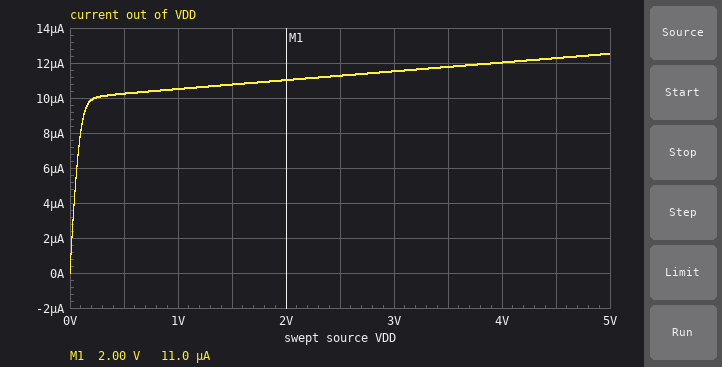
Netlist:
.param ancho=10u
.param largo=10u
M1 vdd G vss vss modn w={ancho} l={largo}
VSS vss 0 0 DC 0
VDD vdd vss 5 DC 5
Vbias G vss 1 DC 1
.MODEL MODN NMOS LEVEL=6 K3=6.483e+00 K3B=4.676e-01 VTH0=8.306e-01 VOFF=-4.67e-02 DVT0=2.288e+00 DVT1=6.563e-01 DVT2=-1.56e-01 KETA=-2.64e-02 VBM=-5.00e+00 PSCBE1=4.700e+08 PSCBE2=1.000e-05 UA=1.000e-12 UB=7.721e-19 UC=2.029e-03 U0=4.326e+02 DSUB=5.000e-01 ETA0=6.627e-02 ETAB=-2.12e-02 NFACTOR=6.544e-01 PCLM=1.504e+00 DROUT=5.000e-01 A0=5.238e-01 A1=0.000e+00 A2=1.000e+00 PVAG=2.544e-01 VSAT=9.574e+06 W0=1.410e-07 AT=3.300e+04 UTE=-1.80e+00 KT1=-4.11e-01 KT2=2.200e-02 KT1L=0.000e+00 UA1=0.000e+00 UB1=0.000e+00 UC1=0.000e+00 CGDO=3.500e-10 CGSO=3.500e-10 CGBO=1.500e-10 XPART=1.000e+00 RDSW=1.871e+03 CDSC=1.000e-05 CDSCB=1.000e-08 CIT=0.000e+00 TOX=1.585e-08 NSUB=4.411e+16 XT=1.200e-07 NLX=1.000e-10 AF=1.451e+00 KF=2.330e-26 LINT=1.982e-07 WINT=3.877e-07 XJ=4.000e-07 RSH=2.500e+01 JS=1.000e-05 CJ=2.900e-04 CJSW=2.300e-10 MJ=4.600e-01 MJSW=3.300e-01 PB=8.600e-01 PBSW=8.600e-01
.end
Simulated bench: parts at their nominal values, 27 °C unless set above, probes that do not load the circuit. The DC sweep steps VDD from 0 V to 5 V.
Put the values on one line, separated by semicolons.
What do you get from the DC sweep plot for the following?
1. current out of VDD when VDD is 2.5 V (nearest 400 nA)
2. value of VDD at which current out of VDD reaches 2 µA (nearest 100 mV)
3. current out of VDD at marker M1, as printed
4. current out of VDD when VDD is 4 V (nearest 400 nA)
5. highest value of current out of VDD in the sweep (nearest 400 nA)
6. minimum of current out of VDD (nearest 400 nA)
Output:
11.2 µA; 0 V; 11.0 µA; 12.0 µA; 12.4 µA; 0 A
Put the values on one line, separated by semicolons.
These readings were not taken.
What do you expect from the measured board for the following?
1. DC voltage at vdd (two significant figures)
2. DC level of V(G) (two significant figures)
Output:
5.0 V; 1.0 V
